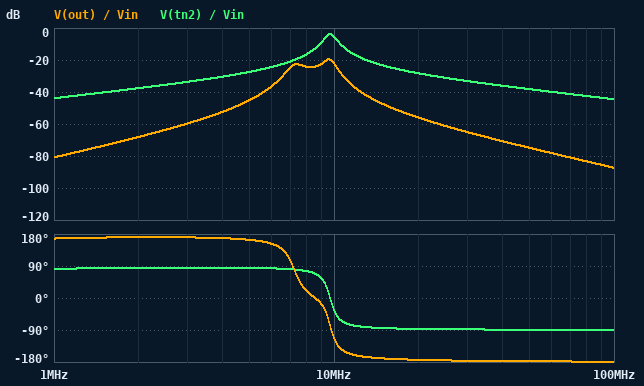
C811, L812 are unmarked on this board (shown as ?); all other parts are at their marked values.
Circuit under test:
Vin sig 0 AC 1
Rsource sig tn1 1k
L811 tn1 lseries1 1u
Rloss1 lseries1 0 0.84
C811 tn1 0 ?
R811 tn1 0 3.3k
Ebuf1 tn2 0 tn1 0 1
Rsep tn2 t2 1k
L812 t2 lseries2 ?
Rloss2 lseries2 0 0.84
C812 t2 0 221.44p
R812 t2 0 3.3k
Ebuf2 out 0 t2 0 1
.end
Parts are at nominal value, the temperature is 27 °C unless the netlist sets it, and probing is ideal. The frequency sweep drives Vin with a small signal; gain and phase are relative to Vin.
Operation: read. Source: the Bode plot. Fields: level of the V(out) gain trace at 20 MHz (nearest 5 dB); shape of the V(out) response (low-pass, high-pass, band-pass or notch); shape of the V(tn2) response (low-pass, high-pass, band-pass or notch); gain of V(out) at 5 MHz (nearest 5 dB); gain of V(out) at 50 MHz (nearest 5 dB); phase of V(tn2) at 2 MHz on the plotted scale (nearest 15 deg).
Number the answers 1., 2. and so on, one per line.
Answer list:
1. -55 dB
2. band-pass
3. band-pass
4. -45 dB
5. -75 dB
6. 90 deg
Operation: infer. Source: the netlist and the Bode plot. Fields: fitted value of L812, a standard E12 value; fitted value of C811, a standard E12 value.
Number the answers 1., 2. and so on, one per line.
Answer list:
1. 2.2 µH
2. 270 pF
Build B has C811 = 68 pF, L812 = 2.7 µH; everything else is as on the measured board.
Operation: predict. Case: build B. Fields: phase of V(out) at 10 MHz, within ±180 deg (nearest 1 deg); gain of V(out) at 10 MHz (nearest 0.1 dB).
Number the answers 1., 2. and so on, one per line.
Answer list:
1. 2 deg
2. -39.6 dB
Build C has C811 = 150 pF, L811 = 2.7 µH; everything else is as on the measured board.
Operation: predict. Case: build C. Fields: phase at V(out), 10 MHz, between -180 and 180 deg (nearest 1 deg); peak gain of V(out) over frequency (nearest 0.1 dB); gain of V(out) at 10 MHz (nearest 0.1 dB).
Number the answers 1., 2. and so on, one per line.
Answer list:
1. -148 deg
2. -7.9 dB
3. -28.2 dB
